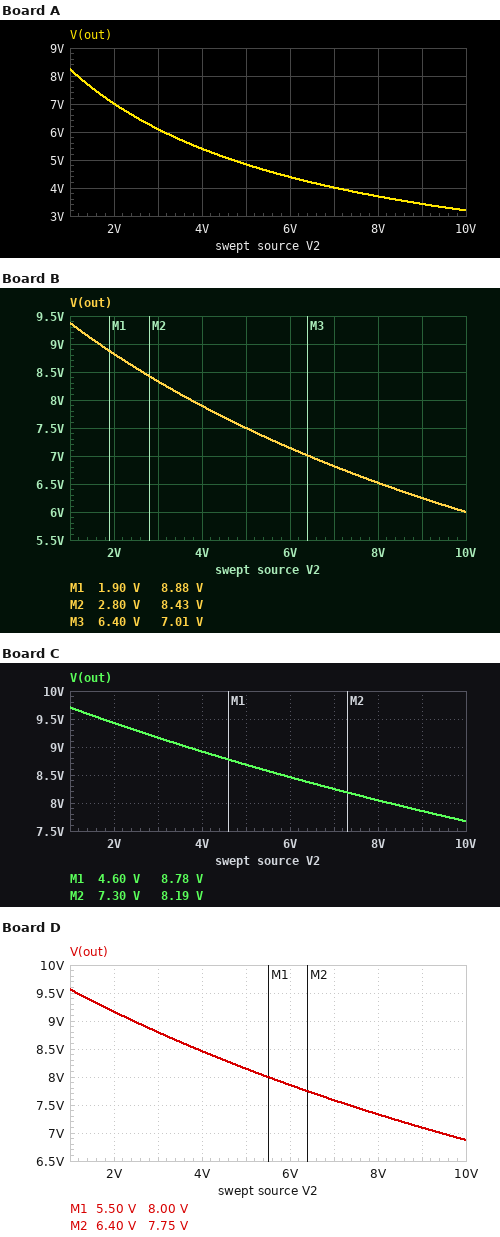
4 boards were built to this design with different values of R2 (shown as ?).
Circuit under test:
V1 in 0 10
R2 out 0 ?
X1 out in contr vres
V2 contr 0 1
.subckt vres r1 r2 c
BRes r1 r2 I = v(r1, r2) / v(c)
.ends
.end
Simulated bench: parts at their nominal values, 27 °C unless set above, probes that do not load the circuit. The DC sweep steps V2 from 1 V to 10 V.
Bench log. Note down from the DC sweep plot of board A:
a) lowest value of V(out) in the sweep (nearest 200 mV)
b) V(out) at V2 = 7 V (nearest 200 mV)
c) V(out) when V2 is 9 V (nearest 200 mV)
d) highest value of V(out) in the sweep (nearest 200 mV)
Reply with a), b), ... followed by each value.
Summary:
a) 3.2 V
b) 4.0 V
c) 3.4 V
d) 8.2 V
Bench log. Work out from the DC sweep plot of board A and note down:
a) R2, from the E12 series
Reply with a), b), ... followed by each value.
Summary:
a) 4.7 Ω
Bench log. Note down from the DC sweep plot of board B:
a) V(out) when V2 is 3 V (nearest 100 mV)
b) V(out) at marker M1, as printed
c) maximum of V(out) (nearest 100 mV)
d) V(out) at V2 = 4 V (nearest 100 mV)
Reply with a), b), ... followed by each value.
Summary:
a) 8.3 V
b) 8.88 V
c) 9.4 V
d) 7.9 V
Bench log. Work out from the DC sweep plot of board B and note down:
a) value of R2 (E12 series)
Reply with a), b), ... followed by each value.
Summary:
a) 15 Ω
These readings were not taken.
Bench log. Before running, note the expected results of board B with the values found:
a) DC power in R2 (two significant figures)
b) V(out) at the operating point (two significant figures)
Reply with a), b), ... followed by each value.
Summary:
a) 5.9 W
b) 9.4 V
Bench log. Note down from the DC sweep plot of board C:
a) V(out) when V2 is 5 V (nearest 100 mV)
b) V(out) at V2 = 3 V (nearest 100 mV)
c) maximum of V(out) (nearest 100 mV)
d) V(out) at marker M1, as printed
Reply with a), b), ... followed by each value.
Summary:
a) 8.7 V
b) 9.2 V
c) 9.7 V
d) 8.78 V
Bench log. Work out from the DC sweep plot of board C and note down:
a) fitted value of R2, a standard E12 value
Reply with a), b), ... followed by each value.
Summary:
a) 33 Ω
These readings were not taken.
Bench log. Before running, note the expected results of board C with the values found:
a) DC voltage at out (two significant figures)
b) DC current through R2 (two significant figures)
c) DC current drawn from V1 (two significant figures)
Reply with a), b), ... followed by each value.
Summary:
a) 9.7 V
b) 290 mA
c) 290 mA
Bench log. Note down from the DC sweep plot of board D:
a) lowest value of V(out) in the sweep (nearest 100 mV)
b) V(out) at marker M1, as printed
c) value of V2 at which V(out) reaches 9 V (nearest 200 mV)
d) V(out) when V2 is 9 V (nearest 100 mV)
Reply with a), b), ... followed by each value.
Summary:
a) 6.9 V
b) 8.00 V
c) 2.4 V
d) 7.1 V
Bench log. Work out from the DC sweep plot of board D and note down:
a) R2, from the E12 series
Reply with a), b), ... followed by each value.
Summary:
a) 22 Ω
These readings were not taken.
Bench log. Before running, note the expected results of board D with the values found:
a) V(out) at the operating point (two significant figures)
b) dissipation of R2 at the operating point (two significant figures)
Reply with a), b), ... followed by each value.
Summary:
a) 9.6 V
b) 4.2 W
